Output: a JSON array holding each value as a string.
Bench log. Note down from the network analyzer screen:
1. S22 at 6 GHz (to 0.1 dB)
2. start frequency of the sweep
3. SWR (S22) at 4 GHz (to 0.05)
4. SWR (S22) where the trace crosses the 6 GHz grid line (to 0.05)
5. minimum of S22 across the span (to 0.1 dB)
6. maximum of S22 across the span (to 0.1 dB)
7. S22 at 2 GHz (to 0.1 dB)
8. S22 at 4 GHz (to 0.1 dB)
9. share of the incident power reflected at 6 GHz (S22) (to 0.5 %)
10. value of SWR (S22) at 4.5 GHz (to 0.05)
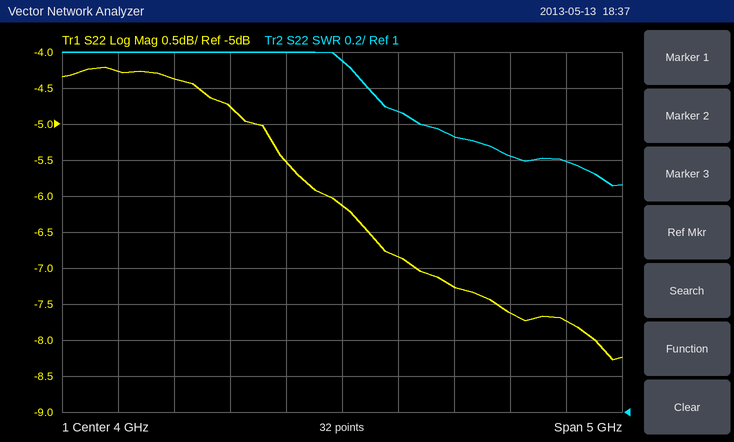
["-7.7 dB", "1.5 GHz", "2.95", "2.40", "-8.3 dB", "-4.2 dB", "-4.3 dB", "-6.1 dB", "17.0 %", "2.65"]
